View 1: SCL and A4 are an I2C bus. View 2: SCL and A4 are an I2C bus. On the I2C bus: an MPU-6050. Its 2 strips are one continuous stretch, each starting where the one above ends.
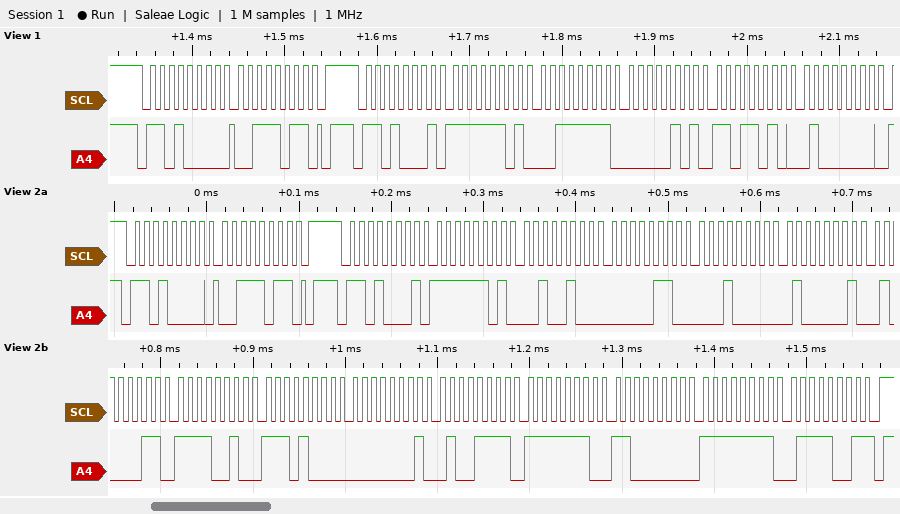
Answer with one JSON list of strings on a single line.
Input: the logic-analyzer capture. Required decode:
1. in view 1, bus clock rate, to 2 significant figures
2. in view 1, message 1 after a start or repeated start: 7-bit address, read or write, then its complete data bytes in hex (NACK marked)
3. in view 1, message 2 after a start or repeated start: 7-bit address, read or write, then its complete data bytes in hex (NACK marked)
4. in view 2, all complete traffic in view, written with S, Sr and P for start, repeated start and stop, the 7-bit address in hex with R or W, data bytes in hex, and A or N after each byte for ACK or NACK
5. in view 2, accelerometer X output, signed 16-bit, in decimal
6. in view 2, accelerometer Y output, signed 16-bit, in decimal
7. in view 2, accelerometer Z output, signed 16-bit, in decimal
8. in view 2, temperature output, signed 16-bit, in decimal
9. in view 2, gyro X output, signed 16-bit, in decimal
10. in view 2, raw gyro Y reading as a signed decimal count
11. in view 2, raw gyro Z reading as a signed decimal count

["100 kHz", "0x68 write: 3B", "0x68 read: FD 3F 05 DA 40", "S 68W A 3B A P S 68R A FD A 24 A 06 A 10 A 41 A 43 A F2 A E8 A 01 A 4F A FE A C0 A FF A 79 N P", "-732", "1552", "16707", "-3352", "335", "-320", "-135"]
